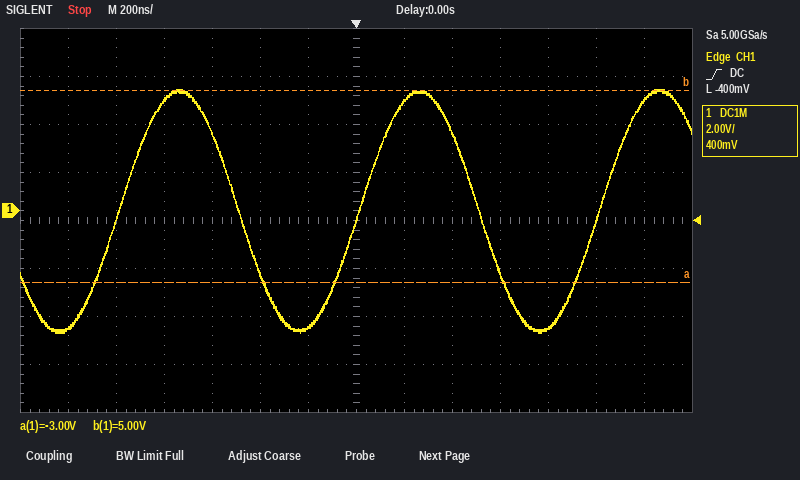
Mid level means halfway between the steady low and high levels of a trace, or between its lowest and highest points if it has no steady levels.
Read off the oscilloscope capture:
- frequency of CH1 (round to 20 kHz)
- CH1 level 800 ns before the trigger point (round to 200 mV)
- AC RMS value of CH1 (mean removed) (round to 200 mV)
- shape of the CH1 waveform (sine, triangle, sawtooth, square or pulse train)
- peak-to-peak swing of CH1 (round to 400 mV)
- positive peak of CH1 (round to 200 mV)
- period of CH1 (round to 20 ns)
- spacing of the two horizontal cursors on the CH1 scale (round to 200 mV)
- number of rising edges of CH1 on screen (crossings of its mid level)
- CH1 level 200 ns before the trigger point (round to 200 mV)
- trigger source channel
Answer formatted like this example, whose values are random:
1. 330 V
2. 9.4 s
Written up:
1. 1.00 MHz
2. 4.6 V
3. 3.6 V
4. sine
5. 10.0 V
6. 5.0 V
7. 1.00 µs
8. 8.0 V
9. 3
10. -4.8 V
11. CH1
